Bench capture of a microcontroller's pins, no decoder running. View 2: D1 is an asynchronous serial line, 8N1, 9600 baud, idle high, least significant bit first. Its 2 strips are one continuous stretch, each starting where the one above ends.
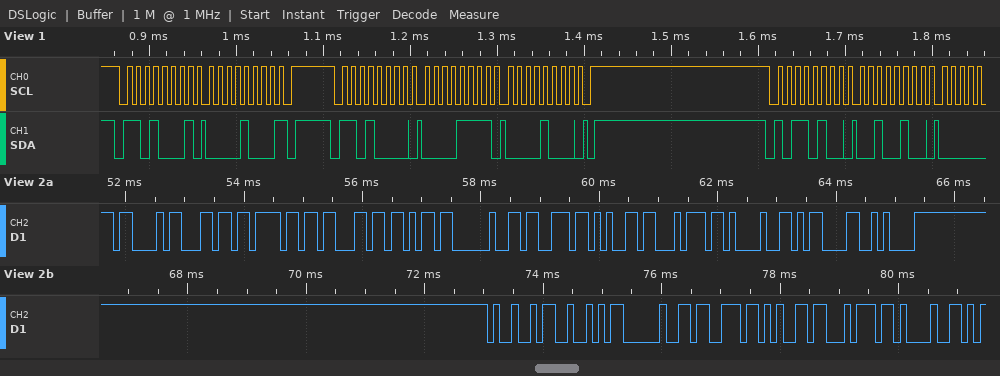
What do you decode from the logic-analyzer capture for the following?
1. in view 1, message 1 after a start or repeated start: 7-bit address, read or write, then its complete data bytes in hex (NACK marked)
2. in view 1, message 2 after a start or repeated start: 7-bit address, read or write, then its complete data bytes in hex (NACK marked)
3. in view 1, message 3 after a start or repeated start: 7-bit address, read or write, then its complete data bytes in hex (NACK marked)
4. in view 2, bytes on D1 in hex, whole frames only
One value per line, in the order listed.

0x68 read: 08 NACK
0x68 write: 0F 08
0x5A write: 24
0x43 0x6C 0x6F 0x63 0x6B 0x20 0x73 0x65 0x74 0x21 0x0D 0x0A 0x49 0x52 0x20 0x73 0x65 0x74 0x21
